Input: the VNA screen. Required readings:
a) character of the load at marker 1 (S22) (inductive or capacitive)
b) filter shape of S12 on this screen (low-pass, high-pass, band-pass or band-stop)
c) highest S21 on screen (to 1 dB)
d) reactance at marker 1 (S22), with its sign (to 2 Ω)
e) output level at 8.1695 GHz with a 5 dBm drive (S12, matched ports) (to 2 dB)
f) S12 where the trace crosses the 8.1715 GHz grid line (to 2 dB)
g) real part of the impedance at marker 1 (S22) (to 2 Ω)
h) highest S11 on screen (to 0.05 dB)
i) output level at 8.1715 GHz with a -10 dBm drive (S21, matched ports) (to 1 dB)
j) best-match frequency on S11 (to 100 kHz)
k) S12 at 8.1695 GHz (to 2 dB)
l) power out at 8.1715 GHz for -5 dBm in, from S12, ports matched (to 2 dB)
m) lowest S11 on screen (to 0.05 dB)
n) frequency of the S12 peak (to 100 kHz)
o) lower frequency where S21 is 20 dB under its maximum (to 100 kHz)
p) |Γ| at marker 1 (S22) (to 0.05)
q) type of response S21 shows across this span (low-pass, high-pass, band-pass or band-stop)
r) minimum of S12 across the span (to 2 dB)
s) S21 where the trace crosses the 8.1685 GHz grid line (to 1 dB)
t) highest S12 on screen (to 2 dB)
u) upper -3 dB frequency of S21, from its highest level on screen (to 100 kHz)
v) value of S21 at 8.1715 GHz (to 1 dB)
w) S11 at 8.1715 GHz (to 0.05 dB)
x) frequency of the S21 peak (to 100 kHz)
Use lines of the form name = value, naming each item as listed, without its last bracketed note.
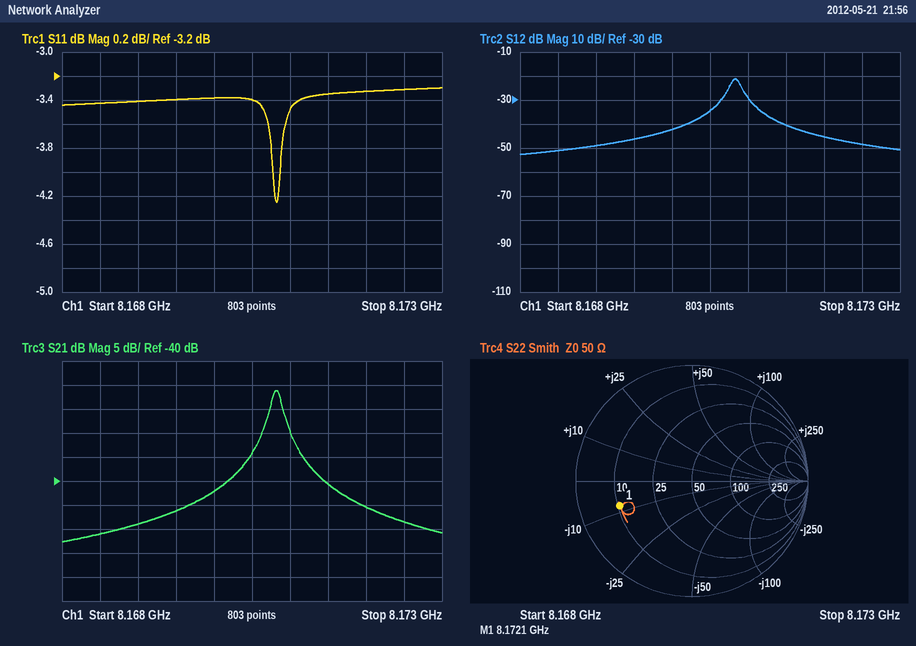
character of the load at marker 1 (S22) = capacitive
filter shape of S12 on this screen = band-pass
highest S21 on screen = -21 dB
reactance at marker 1 (S22), with its sign = -8 Ω
output level at 8.1695 GHz with a 5 dBm drive (S12, matched ports) = -42 dBm
S12 where the trace crosses the 8.1715 GHz grid line = -40 dB
real part of the impedance at marker 1 (S22) = 10 Ω
highest S11 on screen = -3.30 dB
output level at 8.1715 GHz with a -10 dBm drive (S21, matched ports) = -51 dBm
best-match frequency on S11 = 8.1708 GHz
S12 at 8.1695 GHz = -46 dB
power out at 8.1715 GHz for -5 dBm in, from S12, ports matched = -46 dBm
lowest S11 on screen = -4.25 dB
frequency of the S12 peak = 8.1708 GHz
lower frequency where S21 is 20 dB under its maximum = 8.1701 GHz
|Γ| at marker 1 (S22) = 0.65
type of response S21 shows across this span = band-pass
minimum of S12 across the span = -52 dB
S21 where the trace crosses the 8.1685 GHz grid line = -51 dB
highest S12 on screen = -22 dB
upper -3 dB frequency of S21, from its highest level on screen = 8.1709 GHz
value of S21 at 8.1715 GHz = -41 dB
S11 at 8.1715 GHz = -3.35 dB
frequency of the S21 peak = 8.1708 GHz
